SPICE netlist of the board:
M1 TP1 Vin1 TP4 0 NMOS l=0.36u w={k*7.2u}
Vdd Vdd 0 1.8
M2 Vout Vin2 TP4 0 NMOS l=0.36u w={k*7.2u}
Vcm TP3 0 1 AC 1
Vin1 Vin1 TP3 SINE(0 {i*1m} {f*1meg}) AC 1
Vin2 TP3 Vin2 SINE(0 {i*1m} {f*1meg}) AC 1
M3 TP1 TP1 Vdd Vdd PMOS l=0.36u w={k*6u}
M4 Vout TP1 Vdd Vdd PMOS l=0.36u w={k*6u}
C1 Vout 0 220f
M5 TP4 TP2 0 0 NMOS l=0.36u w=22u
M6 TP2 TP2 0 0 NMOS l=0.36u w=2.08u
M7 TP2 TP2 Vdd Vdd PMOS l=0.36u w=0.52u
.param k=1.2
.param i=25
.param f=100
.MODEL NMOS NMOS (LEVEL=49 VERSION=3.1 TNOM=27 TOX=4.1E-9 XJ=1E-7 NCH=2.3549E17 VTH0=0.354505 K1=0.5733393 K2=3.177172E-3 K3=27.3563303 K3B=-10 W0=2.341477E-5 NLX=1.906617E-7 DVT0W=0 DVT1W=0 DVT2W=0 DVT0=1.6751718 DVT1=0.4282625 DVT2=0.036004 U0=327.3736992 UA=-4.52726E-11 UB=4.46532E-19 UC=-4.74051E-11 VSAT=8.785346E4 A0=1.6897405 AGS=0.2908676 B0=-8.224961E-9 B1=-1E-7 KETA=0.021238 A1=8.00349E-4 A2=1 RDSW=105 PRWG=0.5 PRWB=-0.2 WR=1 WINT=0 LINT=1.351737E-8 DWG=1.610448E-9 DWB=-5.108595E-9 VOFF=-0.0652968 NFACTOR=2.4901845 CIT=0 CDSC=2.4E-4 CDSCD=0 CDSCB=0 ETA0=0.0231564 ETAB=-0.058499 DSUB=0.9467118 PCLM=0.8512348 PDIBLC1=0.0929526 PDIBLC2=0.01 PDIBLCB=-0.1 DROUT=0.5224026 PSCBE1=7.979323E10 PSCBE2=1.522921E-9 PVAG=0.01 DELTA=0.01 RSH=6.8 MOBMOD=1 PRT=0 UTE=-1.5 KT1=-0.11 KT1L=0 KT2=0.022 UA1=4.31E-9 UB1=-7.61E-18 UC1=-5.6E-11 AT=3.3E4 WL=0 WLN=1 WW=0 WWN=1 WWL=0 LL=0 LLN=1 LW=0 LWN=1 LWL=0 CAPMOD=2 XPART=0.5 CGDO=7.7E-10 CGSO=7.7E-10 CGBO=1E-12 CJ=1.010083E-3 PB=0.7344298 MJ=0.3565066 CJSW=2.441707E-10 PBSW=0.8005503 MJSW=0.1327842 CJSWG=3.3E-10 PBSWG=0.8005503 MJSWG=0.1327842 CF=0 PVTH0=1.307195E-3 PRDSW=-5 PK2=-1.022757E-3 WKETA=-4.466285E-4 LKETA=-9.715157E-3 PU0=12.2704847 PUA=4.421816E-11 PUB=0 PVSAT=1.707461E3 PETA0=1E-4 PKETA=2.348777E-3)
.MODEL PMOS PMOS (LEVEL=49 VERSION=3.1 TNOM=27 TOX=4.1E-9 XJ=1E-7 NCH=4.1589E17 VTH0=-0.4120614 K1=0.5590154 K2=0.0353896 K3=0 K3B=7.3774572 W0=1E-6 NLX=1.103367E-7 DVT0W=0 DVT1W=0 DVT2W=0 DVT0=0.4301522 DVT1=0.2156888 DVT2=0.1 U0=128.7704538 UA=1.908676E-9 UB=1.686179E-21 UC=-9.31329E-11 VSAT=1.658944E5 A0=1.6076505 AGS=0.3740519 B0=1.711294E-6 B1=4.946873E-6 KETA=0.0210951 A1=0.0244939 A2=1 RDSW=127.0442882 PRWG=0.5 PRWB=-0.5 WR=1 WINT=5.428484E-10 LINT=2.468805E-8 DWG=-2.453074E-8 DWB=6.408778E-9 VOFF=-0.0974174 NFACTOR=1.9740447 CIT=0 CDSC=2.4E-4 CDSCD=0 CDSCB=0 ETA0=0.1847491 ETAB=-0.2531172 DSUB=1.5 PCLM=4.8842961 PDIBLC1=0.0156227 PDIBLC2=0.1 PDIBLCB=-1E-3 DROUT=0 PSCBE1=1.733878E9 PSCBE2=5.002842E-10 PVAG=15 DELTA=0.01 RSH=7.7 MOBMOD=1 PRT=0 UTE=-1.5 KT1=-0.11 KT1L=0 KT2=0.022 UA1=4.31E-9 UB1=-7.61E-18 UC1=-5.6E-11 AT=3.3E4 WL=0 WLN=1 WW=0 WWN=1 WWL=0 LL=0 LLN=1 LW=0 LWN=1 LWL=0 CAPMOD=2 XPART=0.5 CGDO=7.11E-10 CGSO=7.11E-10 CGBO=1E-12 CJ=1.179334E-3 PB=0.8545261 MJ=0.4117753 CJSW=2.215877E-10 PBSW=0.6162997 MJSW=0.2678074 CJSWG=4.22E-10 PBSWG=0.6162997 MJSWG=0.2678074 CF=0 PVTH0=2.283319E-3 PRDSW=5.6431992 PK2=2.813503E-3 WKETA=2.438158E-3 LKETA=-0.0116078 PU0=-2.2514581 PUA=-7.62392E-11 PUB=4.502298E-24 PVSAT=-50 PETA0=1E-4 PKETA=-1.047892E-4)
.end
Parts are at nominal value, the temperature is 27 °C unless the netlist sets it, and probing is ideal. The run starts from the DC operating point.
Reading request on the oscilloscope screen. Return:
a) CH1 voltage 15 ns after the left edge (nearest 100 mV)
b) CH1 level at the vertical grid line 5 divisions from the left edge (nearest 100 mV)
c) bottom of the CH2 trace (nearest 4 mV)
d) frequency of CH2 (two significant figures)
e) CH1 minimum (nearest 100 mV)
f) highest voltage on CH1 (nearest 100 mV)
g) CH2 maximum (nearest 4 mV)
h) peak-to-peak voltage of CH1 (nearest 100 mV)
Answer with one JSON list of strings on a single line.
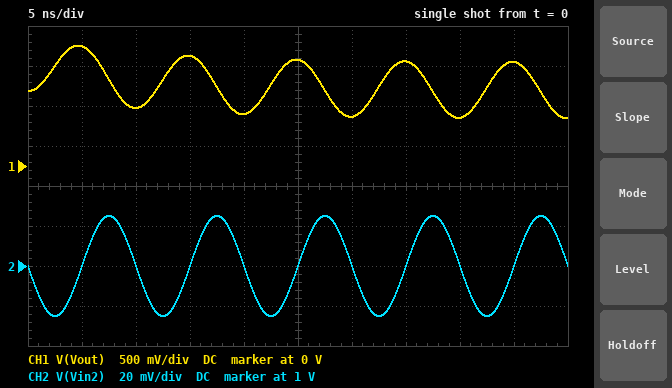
["1.4 V", "1.3 V", "976 mV", "100 MHz", "600 mV", "1.5 V", "1.024 V", "900 mV"]
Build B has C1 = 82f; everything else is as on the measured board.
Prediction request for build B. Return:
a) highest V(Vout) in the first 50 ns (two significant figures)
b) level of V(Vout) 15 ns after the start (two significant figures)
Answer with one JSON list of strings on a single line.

["1.6 V", "1.5 V"]
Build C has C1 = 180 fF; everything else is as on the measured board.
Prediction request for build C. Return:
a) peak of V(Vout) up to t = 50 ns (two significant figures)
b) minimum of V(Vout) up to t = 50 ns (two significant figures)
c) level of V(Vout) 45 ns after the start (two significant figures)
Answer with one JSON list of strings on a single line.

["1.6 V", "530 mV", "1.4 V"]
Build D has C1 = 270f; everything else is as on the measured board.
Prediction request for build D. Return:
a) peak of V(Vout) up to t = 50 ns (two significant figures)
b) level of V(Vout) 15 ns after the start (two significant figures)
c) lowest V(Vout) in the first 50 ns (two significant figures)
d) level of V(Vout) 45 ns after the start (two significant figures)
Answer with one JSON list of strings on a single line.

["1.4 V", "1.3 V", "660 mV", "1.2 V"]
